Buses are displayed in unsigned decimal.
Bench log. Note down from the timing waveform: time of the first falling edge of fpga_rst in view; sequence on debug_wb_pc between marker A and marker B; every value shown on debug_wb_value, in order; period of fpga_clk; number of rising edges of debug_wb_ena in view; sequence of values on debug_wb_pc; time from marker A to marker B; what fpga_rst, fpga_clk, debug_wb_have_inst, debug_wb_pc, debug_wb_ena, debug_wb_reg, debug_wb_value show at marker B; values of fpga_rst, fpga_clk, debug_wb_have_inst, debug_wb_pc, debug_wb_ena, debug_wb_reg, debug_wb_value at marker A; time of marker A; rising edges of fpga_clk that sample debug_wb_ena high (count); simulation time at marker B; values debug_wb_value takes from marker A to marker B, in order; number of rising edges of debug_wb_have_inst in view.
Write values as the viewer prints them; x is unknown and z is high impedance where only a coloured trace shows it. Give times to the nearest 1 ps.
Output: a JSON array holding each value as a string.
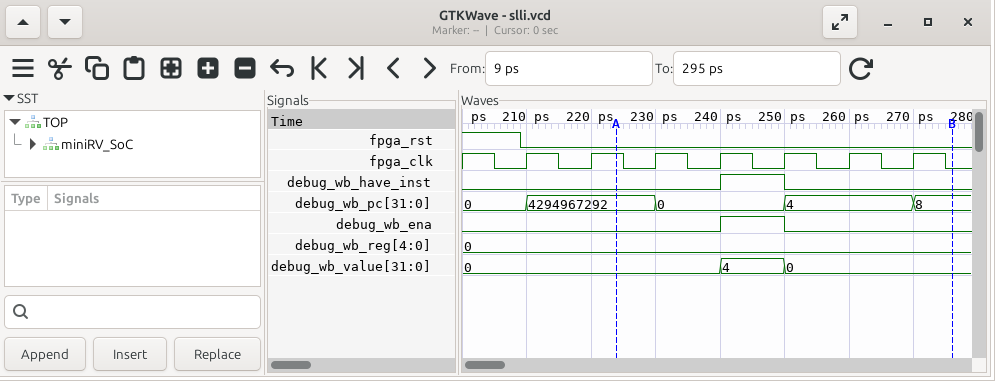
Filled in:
["209 ps", "4294967292, 0, 4, 8", "0, 4, 0", "10 ps", "1", "0, 4294967292, 0, 4, 8", "52 ps", "fpga_rst=0, fpga_clk=0, debug_wb_have_inst=0, debug_wb_pc=8, debug_wb_ena=0, debug_wb_reg=0, debug_wb_value=0", "fpga_rst=0, fpga_clk=1, debug_wb_have_inst=0, debug_wb_pc=4294967292, debug_wb_ena=0, debug_wb_reg=0, debug_wb_value=0", "224 ps", "1", "276 ps", "0, 4, 0", "1"]
